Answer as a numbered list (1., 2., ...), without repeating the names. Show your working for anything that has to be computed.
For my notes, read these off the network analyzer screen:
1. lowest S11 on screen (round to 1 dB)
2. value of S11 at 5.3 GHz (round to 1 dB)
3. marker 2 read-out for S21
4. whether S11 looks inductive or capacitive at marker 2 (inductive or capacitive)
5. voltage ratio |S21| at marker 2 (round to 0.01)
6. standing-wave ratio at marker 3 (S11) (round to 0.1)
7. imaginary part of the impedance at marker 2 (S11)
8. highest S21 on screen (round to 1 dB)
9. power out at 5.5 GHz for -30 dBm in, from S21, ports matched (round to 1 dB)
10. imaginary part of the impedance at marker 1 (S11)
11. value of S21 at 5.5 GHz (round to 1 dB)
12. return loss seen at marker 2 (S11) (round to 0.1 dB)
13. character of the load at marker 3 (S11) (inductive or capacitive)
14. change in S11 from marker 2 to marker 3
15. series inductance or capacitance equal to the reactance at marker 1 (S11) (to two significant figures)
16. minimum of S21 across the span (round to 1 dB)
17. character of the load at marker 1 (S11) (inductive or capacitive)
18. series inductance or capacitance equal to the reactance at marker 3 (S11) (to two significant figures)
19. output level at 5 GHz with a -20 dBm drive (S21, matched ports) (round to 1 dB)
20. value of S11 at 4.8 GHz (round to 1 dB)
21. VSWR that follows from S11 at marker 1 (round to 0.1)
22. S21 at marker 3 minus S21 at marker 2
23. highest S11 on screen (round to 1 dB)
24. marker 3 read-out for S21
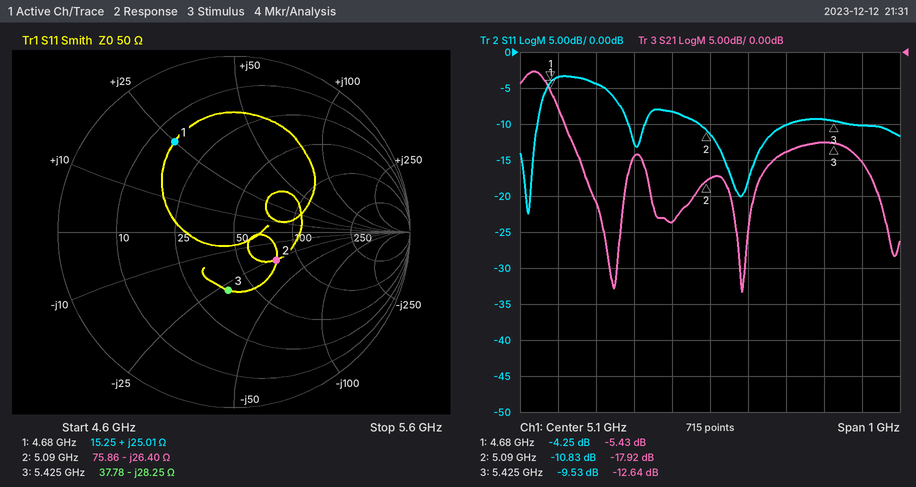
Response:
1. -22 dB
2. -10 dB
3. -17.92 dB
4. capacitive
5. 10^(-17.92/20) ≈ 0.13
6. 2.0
7. -26.40 Ω
8. -3 dB
9. -30 dBm + (-15 dB) = -45 dBm
10. +25.01 Ω
11. -15 dB
12. 10.8 dB
13. capacitive
14. -9.53 − (-10.83) = 1.30 dB
15. L = 25.01 Ω/(2π × 4.68 GHz) ≈ 851 pH, so 850 pH to two significant figures
16. -33 dB
17. inductive
18. C = 1/(2π × 5.425 GHz × 28.25 Ω) ≈ 1.0 pF
19. -20 dBm + (-24 dB) = -44 dBm
20. -4 dB
21. (1 + 0.6131)/(1 − 0.6131) ≈ 4.2
22. -12.64 − (-17.92) = 5.28 dB
23. -3 dB
24. -12.64 dB
